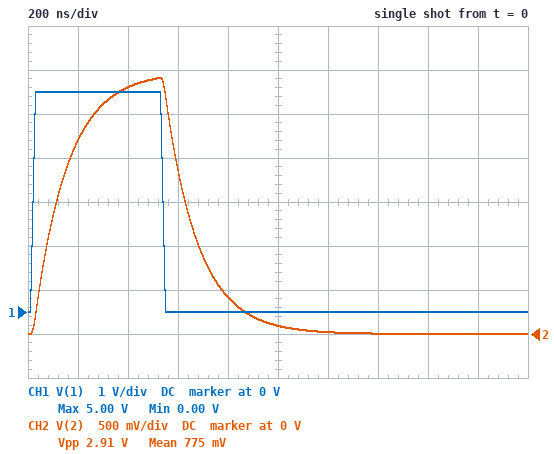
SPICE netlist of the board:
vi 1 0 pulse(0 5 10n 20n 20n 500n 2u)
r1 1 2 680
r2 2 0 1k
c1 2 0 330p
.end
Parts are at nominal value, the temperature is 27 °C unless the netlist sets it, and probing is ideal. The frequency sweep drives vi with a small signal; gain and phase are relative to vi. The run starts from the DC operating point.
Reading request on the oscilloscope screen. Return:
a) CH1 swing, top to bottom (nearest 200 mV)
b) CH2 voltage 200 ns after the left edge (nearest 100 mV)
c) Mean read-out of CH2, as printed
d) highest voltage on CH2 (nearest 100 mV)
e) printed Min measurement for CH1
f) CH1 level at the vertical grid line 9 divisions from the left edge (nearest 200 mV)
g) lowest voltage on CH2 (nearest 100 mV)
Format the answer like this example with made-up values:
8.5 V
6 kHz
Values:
5.0 V
2.2 V
775 mV
2.9 V
0.00 V
0 V
0 V
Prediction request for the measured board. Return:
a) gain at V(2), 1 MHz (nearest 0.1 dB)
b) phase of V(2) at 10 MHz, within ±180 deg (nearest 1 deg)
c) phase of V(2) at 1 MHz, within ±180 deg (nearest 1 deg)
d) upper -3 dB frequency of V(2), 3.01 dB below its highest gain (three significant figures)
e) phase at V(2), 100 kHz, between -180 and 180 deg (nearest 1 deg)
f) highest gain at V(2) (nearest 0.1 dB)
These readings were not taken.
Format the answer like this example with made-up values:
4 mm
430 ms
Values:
-6.8 dB
-83 deg
-40 deg
1.19 MHz
-5 deg
-4.5 dB
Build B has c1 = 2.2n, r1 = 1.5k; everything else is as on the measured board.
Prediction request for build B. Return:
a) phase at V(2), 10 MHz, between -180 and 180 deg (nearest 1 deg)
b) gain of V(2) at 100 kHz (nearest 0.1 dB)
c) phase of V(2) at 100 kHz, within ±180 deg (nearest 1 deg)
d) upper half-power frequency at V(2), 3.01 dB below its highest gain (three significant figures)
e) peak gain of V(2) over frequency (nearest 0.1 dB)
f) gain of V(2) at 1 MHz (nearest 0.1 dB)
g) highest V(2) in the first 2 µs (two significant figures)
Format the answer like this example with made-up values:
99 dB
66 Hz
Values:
-89 deg
-10.2 dB
-40 deg
121 kHz
-8.0 dB
-26.4 dB
650 mV
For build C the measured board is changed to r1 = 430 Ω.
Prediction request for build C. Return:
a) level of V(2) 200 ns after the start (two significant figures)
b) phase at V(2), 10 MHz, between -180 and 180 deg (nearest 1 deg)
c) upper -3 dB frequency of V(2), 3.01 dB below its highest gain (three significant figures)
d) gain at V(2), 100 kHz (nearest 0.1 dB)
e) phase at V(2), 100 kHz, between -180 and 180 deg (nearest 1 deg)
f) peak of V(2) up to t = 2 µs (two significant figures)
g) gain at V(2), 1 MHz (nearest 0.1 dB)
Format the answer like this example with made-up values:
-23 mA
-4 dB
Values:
2.9 V
-81 deg
1.60 MHz
-3.1 dB
-4 deg
3.5 V
-4.5 dB
